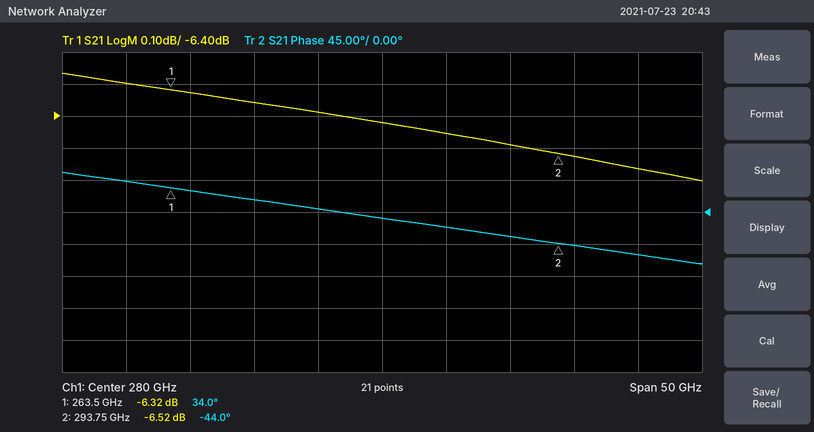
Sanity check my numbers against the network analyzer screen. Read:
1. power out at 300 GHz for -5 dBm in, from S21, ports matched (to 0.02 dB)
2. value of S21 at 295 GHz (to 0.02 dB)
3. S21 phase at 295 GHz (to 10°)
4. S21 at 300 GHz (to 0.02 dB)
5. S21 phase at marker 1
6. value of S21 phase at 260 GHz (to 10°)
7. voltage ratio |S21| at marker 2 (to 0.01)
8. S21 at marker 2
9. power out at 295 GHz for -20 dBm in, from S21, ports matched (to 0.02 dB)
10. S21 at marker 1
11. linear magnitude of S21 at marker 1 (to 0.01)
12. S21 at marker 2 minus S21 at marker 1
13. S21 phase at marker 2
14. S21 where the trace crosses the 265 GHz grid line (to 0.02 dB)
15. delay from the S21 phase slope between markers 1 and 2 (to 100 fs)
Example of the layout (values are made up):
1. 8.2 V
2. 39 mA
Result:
1. -11.56 dBm
2. -6.52 dB
3. -50°
4. -6.56 dB
5. 34.0°
6. 40°
7. 0.47
8. -6.52 dB
9. -26.52 dBm
10. -6.32 dB
11. 0.48
12. -0.20 dB
13. -44.0°
14. -6.32 dB
15. 7.2 ps
